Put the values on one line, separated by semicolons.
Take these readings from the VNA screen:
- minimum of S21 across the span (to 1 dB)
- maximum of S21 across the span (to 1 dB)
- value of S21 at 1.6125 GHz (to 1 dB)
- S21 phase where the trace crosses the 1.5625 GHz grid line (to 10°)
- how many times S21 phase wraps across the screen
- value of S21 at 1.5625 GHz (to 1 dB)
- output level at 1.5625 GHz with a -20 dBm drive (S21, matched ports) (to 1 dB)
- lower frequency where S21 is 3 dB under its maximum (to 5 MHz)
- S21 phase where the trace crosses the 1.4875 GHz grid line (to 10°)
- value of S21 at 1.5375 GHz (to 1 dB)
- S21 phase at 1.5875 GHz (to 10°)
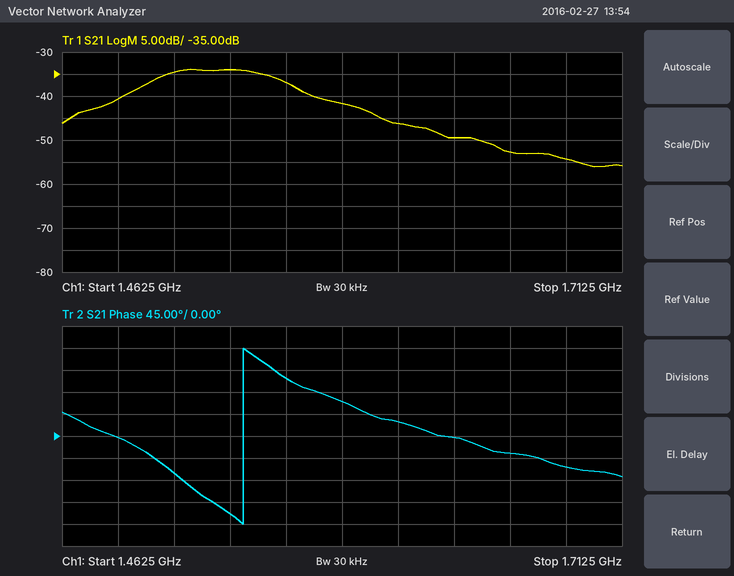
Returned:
-56 dB; -34 dB; -46 dB; 120°; 1; -37 dB; -57 dBm; 1.500 GHz; 0°; -34 dB; 70°
